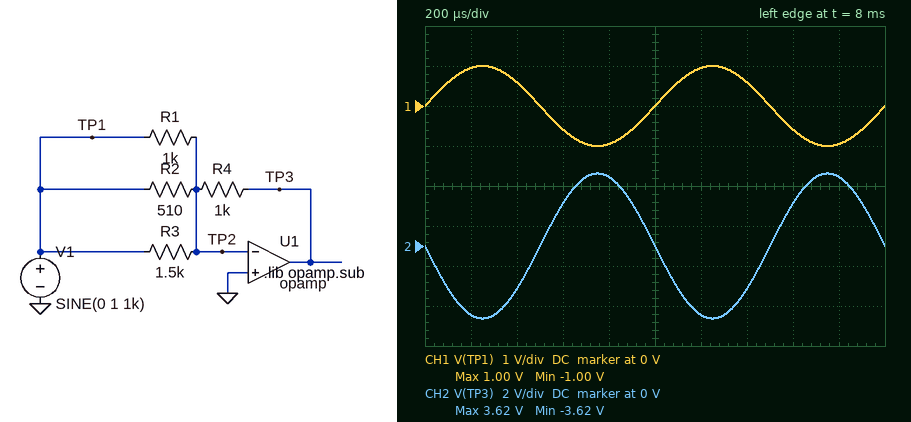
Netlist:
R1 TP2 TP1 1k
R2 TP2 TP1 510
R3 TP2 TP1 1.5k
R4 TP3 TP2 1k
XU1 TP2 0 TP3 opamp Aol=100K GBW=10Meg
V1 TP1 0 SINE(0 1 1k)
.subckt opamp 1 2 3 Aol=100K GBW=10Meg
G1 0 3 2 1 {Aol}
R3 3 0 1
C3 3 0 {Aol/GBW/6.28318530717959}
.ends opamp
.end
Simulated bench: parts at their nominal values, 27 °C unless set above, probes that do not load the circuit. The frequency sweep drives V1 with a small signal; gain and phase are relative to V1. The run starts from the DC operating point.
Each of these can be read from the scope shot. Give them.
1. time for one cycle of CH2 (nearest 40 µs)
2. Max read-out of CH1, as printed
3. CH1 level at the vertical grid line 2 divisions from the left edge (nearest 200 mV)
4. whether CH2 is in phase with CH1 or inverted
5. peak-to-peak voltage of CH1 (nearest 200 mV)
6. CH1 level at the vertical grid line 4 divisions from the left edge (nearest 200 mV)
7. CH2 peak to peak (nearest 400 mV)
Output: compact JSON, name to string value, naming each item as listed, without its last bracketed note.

{"time for one cycle of CH2": "1.00 ms", "Max read-out of CH1, as printed": "1.00 V", "CH1 level at the vertical grid line 2 divisions from the left edge": "600 mV", "whether CH2 is in phase with CH1 or inverted": "inverted", "peak-to-peak voltage of CH1": "2.0 V", "CH1 level at the vertical grid line 4 divisions from the left edge": "-1.0 V", "CH2 peak to peak": "7.2 V"}
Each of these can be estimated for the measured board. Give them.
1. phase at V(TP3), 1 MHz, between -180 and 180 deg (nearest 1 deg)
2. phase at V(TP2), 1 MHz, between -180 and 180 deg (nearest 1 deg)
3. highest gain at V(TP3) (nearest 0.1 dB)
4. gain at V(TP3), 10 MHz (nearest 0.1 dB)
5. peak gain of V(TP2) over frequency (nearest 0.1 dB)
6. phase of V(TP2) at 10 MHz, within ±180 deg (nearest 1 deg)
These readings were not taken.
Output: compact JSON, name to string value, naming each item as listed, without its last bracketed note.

{"phase at V(TP3), 1 MHz, between -180 and 180 deg": "155 deg", "phase at V(TP2), 1 MHz, between -180 and 180 deg": "65 deg", "highest gain at V(TP3)": "11.2 dB", "gain at V(TP3), 10 MHz": "-2.3 dB", "peak gain of V(TP2) over frequency": "-2.1 dB", "phase of V(TP2) at 10 MHz, within ±180 deg": "12 deg"}
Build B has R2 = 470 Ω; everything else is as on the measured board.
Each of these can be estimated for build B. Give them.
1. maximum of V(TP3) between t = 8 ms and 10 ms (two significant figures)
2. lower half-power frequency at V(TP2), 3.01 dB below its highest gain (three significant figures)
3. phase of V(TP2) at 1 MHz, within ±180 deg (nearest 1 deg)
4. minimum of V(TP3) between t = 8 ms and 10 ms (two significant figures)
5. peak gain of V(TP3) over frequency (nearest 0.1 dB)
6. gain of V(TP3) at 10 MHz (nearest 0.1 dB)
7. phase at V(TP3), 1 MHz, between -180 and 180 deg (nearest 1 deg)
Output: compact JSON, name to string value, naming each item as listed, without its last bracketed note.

{"maximum of V(TP3) between t = 8 ms and 10 ms": "3.8 V", "lower half-power frequency at V(TP2), 3.01 dB below its highest gain": "2.09 MHz", "phase of V(TP2) at 1 MHz, within ±180 deg": "64 deg", "minimum of V(TP3) between t = 8 ms and 10 ms": "-3.8 V", "peak gain of V(TP3) over frequency": "11.6 dB", "gain of V(TP3) at 10 MHz": "-2.2 dB", "phase at V(TP3), 1 MHz, between -180 and 180 deg": "154 deg"}
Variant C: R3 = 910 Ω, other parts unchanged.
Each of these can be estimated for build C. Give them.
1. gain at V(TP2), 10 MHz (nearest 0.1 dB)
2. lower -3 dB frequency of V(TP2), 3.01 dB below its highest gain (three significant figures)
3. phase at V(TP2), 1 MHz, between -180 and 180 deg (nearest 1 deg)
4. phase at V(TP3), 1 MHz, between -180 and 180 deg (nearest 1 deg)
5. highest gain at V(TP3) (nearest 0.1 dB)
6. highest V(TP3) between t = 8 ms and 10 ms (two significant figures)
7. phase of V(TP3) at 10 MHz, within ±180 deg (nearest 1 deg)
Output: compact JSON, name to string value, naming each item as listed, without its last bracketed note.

{"gain at V(TP2), 10 MHz": "-2.1 dB", "lower -3 dB frequency of V(TP2), 3.01 dB below its highest gain": "1.98 MHz", "phase at V(TP2), 1 MHz, between -180 and 180 deg": "63 deg", "phase at V(TP3), 1 MHz, between -180 and 180 deg": "153 deg", "highest gain at V(TP3)": "12.2 dB", "highest V(TP3) between t = 8 ms and 10 ms": "4.1 V", "phase of V(TP3) at 10 MHz, within ±180 deg": "101 deg"}
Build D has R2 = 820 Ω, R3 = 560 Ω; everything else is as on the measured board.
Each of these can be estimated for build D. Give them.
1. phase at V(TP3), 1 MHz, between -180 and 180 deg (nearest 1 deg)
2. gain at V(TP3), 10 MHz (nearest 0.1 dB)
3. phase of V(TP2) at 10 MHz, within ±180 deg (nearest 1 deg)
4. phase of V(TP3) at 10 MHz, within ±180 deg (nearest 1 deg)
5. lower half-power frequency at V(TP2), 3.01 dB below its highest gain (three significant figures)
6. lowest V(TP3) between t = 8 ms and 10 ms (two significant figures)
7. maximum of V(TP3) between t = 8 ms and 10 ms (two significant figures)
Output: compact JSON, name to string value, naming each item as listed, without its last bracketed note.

{"phase at V(TP3), 1 MHz, between -180 and 180 deg": "153 deg", "gain at V(TP3), 10 MHz": "-2.1 dB", "phase of V(TP2) at 10 MHz, within ±180 deg": "11 deg", "phase of V(TP3) at 10 MHz, within ±180 deg": "101 deg", "lower half-power frequency at V(TP2), 3.01 dB below its highest gain": "2.00 MHz", "lowest V(TP3) between t = 8 ms and 10 ms": "-4.0 V", "maximum of V(TP3) between t = 8 ms and 10 ms": "4.0 V"}
